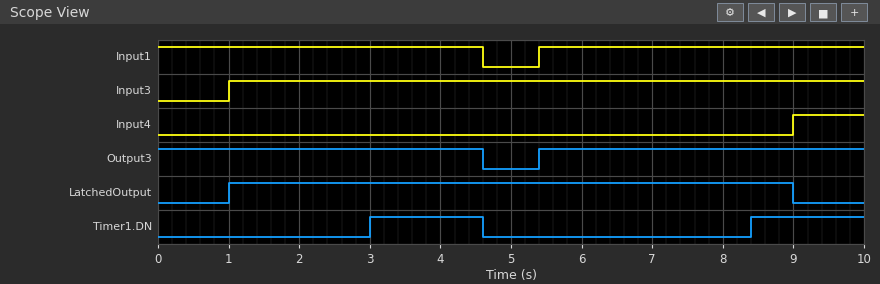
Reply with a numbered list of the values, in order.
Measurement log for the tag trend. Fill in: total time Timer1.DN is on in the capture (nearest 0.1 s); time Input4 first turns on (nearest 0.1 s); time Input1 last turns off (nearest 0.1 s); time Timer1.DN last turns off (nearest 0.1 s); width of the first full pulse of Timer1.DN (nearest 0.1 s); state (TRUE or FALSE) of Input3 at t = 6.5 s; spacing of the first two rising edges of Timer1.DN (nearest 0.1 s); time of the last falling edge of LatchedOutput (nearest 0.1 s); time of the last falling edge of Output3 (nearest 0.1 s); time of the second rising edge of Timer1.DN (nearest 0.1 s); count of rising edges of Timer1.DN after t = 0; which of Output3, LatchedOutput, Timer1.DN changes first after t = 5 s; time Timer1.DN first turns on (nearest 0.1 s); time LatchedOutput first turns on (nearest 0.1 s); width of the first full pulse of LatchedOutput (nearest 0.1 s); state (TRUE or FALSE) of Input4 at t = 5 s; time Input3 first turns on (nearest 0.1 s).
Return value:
1. 3.2 s
2. 9.0 s
3. 4.6 s
4. 4.6 s
5. 1.6 s
6. TRUE
7. 5.4 s
8. 9.0 s
9. 4.6 s
10. 8.4 s
11. 2
12. Output3
13. 3.0 s
14. 1.0 s
15. 8.0 s
16. FALSE
17. 1.0 s
